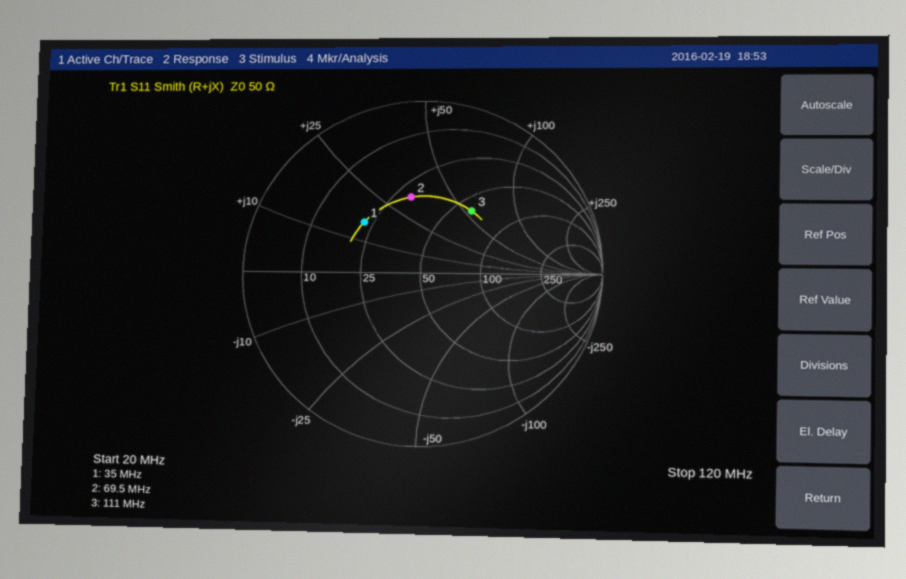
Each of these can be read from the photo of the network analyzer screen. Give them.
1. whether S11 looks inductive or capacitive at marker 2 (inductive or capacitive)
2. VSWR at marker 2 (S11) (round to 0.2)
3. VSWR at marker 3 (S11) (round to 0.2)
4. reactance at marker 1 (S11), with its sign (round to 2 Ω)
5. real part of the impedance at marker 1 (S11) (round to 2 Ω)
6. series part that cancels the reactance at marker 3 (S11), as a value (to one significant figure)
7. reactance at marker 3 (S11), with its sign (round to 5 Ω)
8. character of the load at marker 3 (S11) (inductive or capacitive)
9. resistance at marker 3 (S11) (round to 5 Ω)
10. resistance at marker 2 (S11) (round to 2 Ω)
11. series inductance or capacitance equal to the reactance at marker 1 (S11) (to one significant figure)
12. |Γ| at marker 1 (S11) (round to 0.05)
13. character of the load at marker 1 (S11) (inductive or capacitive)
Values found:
inductive
2.6
2.6
+16 Ω
22 Ω
30 pF
+55 Ω
inductive
60 Ω
30 Ω
70 nH
0.45
inductive
